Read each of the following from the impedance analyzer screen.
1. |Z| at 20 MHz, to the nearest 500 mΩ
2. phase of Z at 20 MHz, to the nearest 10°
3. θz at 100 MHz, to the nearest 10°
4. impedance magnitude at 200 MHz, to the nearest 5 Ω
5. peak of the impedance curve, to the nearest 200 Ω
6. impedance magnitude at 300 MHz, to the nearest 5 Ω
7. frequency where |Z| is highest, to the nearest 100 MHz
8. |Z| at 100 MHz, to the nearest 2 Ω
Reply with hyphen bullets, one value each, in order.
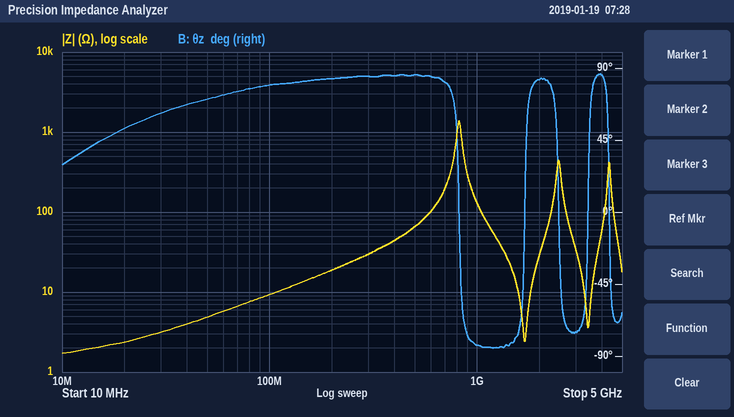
- 2.5 Ω
- 50°
- 80°
- 20 Ω
- 1.4 kΩ
- 30 Ω
- 800 MHz
- 10 Ω
